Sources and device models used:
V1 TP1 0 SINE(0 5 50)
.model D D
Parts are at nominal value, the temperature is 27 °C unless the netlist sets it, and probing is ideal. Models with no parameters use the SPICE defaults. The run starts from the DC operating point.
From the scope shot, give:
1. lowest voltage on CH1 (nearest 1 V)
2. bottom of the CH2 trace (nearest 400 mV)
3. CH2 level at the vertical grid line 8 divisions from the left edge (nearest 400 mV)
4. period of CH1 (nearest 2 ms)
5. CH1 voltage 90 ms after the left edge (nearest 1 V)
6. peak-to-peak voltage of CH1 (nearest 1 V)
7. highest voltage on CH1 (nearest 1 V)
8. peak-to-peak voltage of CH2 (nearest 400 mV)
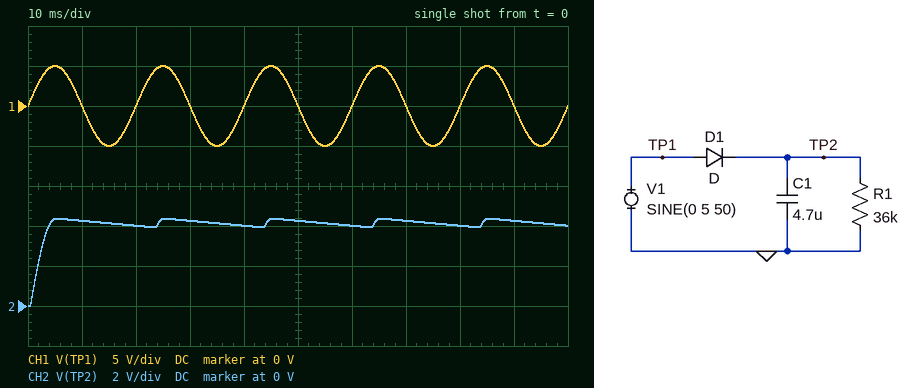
-5 V
0 V
4.0 V
20 ms
0 V
10 V
5 V
4.4 V
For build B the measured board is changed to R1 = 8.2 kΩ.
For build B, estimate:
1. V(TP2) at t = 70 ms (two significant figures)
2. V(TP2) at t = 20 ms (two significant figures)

3.9 V
3.0 V
